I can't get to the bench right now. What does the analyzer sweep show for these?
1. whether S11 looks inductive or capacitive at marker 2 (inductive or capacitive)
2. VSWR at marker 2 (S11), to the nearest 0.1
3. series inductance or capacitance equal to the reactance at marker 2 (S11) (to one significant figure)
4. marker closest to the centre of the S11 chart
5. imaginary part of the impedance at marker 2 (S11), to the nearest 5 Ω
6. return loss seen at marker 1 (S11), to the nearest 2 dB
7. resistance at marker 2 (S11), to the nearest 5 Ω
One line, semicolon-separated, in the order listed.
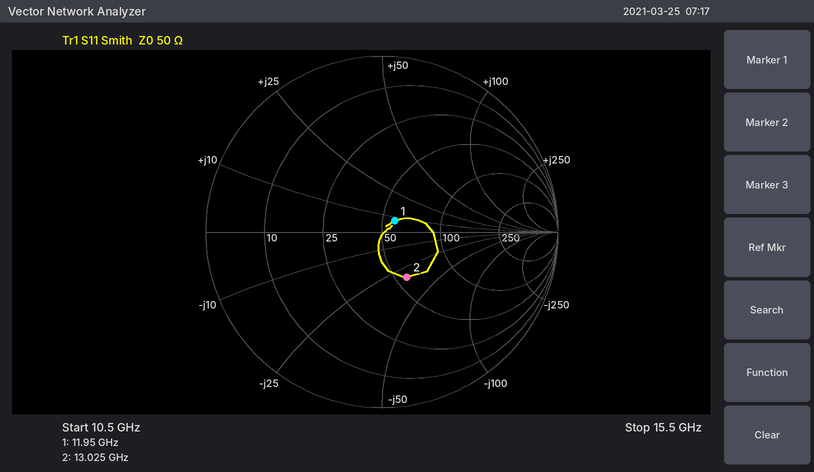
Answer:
capacitive; 1.8; 400 fF; marker 1; -30 Ω; 20 dB; 55 Ω
